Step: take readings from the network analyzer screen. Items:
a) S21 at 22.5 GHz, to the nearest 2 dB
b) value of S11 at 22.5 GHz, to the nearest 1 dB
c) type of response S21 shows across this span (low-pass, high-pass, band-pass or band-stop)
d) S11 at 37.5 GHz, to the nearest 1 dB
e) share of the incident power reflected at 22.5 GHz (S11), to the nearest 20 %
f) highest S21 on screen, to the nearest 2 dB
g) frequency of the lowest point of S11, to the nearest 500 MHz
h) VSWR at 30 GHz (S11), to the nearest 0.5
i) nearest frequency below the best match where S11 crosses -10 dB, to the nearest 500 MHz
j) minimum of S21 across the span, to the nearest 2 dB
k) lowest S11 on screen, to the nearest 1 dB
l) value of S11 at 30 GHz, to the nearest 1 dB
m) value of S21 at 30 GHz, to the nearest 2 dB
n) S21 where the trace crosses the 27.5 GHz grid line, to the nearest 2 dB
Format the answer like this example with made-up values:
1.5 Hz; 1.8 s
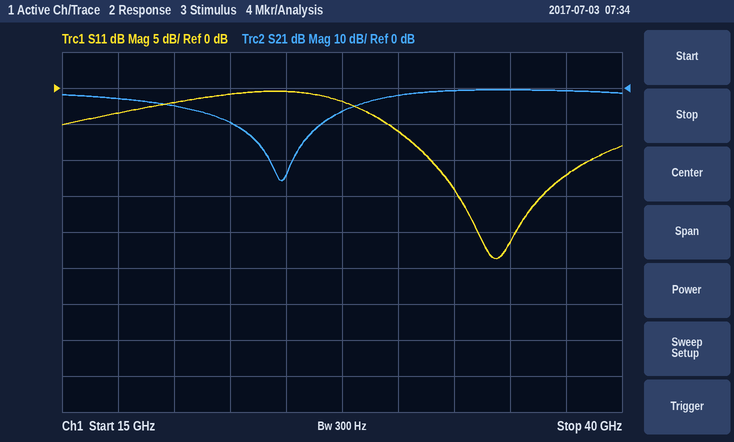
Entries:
-10 dB; -1 dB; band-stop; -12 dB; 80 %; 0 dB; 34.5 GHz; 3.0; 31.5 GHz; -26 dB; -24 dB; -6 dB; -2 dB; -6 dB
